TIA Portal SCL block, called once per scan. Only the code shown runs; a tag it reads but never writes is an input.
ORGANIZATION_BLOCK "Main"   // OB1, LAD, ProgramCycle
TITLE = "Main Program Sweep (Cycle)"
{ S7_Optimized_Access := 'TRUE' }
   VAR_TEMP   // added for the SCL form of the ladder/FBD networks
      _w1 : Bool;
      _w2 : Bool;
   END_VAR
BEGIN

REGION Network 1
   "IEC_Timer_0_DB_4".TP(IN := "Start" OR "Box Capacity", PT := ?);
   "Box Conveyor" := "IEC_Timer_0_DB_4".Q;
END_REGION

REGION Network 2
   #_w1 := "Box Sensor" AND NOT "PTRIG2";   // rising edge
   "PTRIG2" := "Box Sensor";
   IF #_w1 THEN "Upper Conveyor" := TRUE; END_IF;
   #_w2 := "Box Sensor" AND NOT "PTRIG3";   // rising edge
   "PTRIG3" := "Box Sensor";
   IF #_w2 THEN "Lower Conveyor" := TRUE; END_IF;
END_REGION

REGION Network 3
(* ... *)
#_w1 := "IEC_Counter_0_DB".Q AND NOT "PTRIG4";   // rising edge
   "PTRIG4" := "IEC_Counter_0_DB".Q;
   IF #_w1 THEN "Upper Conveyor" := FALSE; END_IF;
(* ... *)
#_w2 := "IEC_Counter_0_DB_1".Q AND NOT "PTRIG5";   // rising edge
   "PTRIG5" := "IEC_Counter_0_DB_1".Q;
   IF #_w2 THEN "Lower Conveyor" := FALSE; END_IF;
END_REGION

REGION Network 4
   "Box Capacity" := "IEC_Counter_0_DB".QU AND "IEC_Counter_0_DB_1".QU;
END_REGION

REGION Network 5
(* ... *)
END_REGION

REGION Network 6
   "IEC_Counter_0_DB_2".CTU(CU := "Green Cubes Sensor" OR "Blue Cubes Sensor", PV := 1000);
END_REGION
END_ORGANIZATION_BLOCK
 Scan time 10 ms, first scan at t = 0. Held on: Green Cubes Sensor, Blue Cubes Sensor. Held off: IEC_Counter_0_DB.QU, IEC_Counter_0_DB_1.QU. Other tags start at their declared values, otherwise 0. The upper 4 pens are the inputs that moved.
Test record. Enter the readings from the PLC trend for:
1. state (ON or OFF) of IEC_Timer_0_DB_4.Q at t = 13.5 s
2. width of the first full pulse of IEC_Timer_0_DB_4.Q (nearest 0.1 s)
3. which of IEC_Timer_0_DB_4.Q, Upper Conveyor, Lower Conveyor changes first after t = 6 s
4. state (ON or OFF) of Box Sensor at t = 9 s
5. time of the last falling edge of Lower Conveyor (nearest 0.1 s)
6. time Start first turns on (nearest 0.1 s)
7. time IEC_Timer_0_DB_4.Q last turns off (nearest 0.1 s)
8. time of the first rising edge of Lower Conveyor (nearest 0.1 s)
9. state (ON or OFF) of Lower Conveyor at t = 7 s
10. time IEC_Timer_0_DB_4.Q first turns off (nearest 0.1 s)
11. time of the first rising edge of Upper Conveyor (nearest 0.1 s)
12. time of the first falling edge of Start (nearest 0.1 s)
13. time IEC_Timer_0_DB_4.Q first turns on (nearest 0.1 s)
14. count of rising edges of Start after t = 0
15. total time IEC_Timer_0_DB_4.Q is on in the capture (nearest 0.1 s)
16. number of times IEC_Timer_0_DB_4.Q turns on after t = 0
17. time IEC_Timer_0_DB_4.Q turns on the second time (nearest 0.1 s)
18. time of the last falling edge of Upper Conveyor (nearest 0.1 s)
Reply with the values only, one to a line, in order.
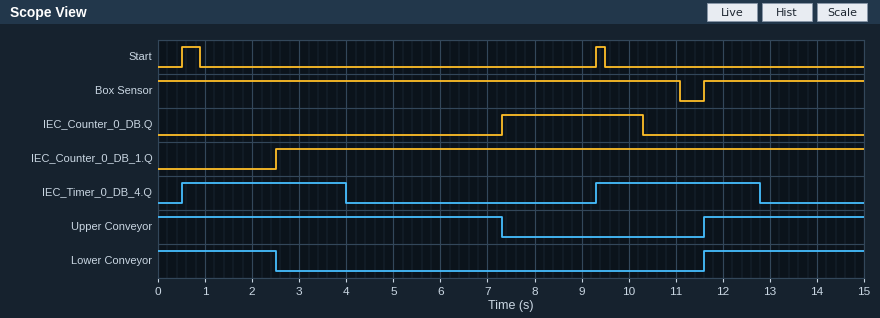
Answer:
OFF
3.5 s
Upper Conveyor
ON
2.5 s
0.5 s
12.8 s
11.6 s
OFF
4.0 s
11.6 s
0.9 s
0.5 s
2
7.0 s
2
9.3 s
7.3 s
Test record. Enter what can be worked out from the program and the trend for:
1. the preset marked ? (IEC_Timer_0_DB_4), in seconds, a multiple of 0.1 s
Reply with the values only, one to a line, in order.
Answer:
3.5 s
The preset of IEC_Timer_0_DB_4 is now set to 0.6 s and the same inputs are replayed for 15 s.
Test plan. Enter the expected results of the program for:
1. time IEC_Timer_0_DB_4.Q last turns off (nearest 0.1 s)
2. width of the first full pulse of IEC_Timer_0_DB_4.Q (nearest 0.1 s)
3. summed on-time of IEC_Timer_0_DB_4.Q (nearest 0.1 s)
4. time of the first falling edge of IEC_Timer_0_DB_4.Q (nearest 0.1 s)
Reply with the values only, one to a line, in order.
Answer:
9.9 s
0.6 s
1.2 s
1.1 s
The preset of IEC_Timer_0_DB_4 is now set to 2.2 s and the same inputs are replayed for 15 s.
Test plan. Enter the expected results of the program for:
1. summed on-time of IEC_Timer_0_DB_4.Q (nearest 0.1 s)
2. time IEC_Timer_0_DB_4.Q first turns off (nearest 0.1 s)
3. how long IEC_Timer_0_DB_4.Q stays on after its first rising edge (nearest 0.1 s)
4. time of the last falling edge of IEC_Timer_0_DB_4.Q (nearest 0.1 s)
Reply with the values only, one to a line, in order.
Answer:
4.4 s
2.7 s
2.2 s
11.5 s
